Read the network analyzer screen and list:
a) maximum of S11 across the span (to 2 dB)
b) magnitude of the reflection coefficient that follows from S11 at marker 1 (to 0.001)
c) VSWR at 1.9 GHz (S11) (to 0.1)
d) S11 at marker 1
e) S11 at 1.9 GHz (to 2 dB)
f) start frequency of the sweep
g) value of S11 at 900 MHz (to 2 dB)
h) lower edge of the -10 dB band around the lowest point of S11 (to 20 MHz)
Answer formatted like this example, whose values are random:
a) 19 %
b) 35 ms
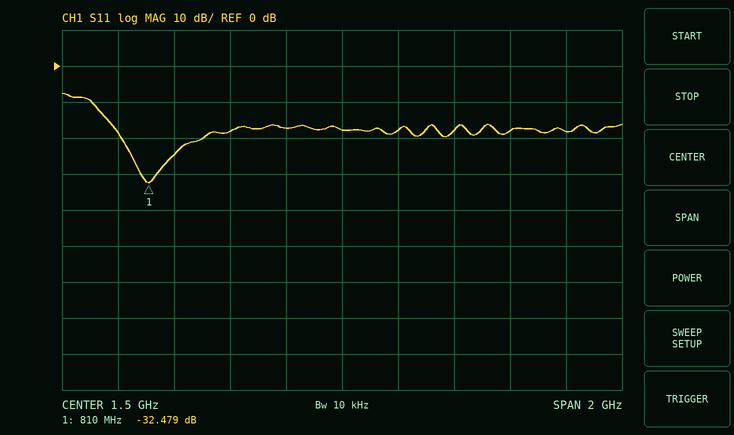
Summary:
a) -8 dB
b) 0.024
c) 1.3
d) -32.479 dB
e) -18 dB
f) 500 MHz
g) -24 dB
h) 600 MHz
